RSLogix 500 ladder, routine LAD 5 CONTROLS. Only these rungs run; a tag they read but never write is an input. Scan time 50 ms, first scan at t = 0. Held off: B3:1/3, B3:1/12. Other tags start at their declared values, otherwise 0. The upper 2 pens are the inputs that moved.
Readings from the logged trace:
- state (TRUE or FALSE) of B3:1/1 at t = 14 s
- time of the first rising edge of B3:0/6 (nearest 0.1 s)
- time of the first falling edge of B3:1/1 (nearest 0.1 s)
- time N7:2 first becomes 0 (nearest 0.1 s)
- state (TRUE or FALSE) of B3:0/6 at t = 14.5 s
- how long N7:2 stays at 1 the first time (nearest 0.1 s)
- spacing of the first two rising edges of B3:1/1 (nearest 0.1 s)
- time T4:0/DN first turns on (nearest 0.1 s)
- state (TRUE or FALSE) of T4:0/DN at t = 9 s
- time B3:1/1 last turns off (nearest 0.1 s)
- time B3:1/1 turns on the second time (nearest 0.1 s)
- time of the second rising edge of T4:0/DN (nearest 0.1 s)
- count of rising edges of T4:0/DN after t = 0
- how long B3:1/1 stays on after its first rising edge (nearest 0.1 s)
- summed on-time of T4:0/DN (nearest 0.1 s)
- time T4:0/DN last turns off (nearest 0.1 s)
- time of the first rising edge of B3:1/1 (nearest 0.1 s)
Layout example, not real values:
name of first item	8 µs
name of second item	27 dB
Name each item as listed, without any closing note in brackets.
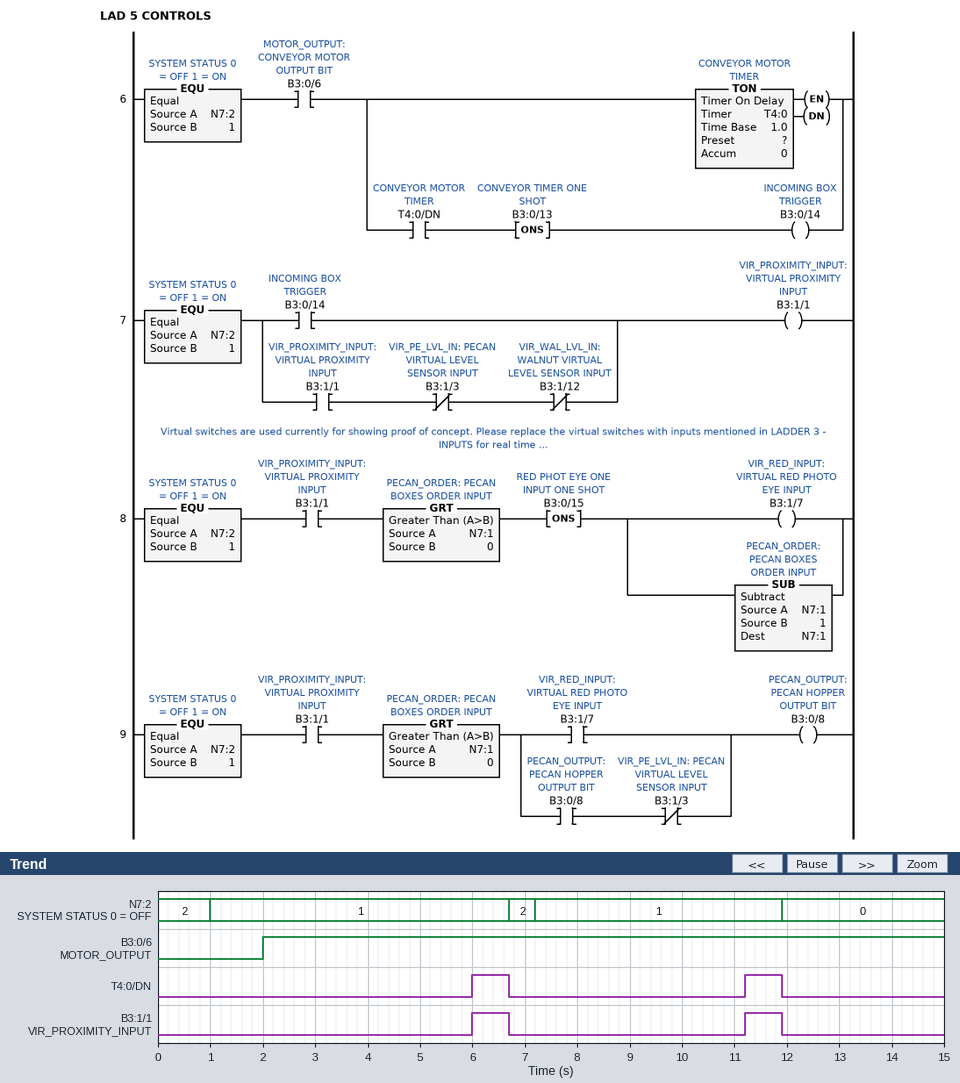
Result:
state (TRUE or FALSE) of B3:1/1 at t = 14 s	FALSE
time of the first rising edge of B3:0/6	2.0 s
time of the first falling edge of B3:1/1	6.7 s
time N7:2 first becomes 0	11.9 s
state (TRUE or FALSE) of B3:0/6 at t = 14.5 s	TRUE
how long N7:2 stays at 1 the first time	5.7 s
spacing of the first two rising edges of B3:1/1	5.2 s
time T4:0/DN first turns on	6.0 s
state (TRUE or FALSE) of T4:0/DN at t = 9 s	FALSE
time B3:1/1 last turns off	11.9 s
time B3:1/1 turns on the second time	11.2 s
time of the second rising edge of T4:0/DN	11.2 s
count of rising edges of T4:0/DN after t = 0	2
how long B3:1/1 stays on after its first rising edge	0.7 s
summed on-time of T4:0/DN	1.4 s
time T4:0/DN last turns off	11.9 s
time of the first rising edge of B3:1/1	6.0 s
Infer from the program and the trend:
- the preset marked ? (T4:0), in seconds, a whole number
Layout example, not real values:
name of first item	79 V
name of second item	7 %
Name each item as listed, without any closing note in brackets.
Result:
the preset marked ? (T4:0), in seconds, a whole number	4 s
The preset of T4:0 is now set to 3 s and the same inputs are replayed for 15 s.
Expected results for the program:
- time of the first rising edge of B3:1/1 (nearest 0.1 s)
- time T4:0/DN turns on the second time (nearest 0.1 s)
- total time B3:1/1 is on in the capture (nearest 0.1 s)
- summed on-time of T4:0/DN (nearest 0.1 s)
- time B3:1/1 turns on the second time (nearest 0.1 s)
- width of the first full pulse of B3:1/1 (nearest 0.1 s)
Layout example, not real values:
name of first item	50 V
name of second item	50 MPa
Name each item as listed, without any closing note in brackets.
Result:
time of the first rising edge of B3:1/1	5.0 s
time T4:0/DN turns on the second time	10.2 s
total time B3:1/1 is on in the capture	3.4 s
summed on-time of T4:0/DN	3.4 s
time B3:1/1 turns on the second time	10.2 s
width of the first full pulse of B3:1/1	1.7 s
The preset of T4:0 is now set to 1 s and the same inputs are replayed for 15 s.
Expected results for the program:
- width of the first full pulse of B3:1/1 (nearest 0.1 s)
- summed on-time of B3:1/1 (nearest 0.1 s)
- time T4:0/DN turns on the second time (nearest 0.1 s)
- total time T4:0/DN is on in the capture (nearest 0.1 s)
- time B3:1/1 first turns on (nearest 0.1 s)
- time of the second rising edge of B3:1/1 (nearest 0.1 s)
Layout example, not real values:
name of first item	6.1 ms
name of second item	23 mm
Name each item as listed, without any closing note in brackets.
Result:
width of the first full pulse of B3:1/1	3.7 s
summed on-time of B3:1/1	7.4 s
time T4:0/DN turns on the second time	8.2 s
total time T4:0/DN is on in the capture	7.4 s
time B3:1/1 first turns on	3.0 s
time of the second rising edge of B3:1/1	8.2 s
